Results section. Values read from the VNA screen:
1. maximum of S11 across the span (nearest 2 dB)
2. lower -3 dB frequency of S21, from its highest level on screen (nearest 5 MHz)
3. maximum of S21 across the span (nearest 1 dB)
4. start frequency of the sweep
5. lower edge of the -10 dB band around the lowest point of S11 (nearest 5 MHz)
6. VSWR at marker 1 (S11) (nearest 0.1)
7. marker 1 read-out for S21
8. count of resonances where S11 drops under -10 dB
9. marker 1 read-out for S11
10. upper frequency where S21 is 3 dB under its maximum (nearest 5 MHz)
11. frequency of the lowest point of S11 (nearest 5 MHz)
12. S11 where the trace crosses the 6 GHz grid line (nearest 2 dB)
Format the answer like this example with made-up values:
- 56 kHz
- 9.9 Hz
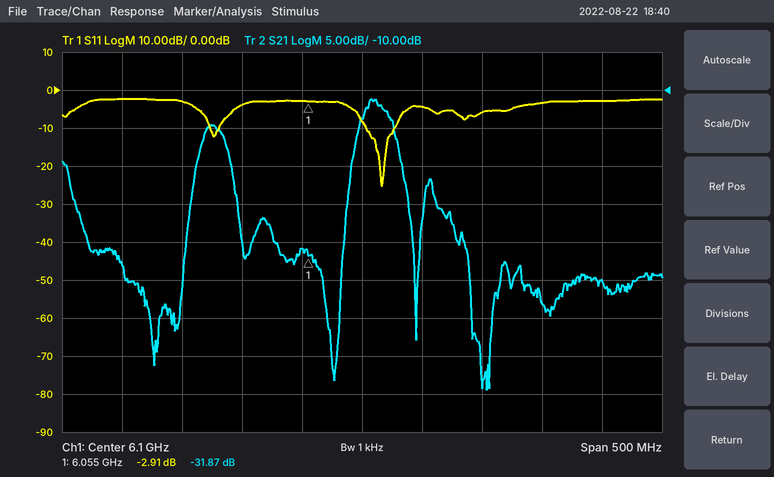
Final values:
- -2 dB
- 6.100 GHz
- -11 dB
- 5.85 GHz
- 6.105 GHz
- 6.0
- -31.87 dB
- 2
- -2.91 dB
- 6.125 GHz
- 6.115 GHz
- -4 dB
